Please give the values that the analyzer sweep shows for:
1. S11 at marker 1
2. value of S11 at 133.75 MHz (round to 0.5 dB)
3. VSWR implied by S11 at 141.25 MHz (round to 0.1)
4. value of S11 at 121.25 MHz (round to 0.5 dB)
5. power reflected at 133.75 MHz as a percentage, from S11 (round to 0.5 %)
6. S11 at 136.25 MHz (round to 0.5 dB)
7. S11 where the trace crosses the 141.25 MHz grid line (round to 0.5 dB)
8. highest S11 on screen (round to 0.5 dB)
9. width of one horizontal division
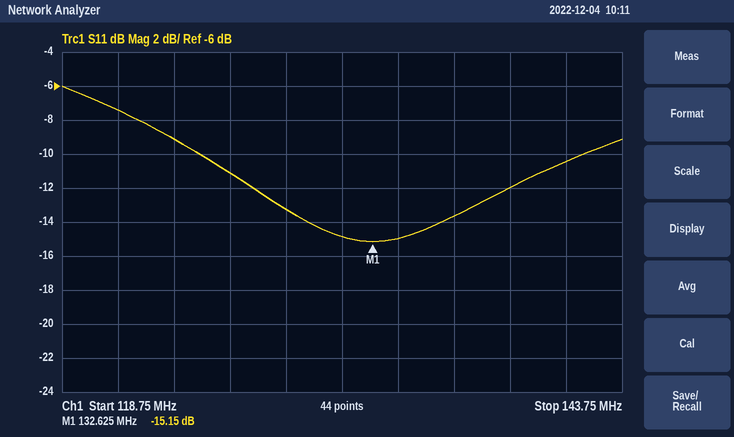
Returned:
-15.15 dB
-15.0 dB
1.9
-7.5 dB
3.0 %
-13.5 dB
-10.5 dB
-6.0 dB
2.5 MHz
